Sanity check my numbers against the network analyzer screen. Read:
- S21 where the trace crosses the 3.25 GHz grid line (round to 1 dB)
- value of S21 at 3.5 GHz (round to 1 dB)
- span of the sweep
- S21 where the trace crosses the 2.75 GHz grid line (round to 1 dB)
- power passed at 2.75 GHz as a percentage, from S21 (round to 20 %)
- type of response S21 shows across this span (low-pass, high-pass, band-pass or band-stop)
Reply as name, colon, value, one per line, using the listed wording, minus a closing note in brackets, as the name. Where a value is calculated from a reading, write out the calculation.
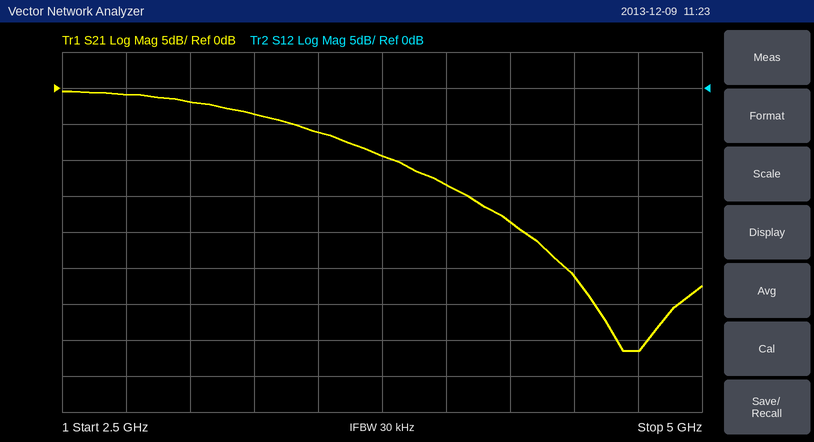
S21 where the trace crosses the 3.25 GHz grid line: -4 dB
value of S21 at 3.5 GHz: -6 dB
span of the sweep: 2.5 GHz
S21 where the trace crosses the 2.75 GHz grid line: -1 dB
power passed at 2.75 GHz as a percentage, from S21: 10^(-1/10) ≈ 79.4 %, so 80 % to the nearest 20 %
type of response S21 shows across this span: low-pass
